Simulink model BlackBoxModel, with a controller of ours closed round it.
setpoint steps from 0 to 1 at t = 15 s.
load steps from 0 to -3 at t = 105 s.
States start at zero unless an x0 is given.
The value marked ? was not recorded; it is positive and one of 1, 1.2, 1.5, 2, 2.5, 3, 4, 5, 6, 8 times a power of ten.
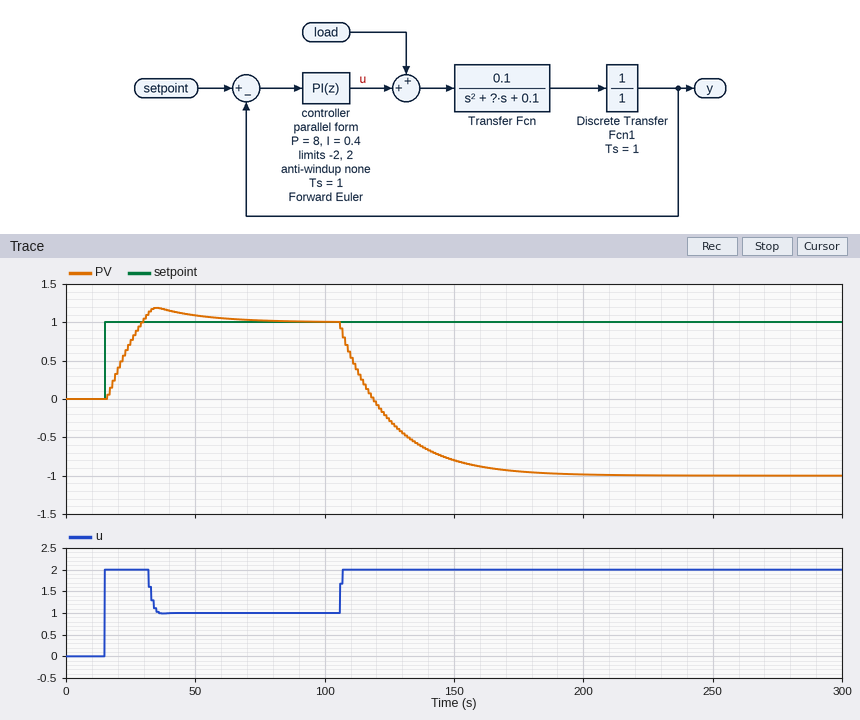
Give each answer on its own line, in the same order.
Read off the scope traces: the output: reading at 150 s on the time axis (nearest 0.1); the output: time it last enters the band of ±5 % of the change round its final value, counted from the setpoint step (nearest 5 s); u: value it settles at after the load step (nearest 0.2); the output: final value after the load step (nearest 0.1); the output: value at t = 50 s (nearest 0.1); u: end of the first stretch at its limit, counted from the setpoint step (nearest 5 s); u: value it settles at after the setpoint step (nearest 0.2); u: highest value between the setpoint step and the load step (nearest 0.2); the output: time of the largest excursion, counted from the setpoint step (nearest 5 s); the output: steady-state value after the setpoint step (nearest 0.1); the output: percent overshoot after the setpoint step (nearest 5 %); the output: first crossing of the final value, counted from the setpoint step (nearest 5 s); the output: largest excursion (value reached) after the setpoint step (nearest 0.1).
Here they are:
-0.8
45 s
2.0
-1.0
1.1
15 s
1.0
2.0
20 s
1.0
20 %
15 s
1.2
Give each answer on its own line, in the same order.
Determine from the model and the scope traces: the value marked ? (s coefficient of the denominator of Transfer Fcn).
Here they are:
2
